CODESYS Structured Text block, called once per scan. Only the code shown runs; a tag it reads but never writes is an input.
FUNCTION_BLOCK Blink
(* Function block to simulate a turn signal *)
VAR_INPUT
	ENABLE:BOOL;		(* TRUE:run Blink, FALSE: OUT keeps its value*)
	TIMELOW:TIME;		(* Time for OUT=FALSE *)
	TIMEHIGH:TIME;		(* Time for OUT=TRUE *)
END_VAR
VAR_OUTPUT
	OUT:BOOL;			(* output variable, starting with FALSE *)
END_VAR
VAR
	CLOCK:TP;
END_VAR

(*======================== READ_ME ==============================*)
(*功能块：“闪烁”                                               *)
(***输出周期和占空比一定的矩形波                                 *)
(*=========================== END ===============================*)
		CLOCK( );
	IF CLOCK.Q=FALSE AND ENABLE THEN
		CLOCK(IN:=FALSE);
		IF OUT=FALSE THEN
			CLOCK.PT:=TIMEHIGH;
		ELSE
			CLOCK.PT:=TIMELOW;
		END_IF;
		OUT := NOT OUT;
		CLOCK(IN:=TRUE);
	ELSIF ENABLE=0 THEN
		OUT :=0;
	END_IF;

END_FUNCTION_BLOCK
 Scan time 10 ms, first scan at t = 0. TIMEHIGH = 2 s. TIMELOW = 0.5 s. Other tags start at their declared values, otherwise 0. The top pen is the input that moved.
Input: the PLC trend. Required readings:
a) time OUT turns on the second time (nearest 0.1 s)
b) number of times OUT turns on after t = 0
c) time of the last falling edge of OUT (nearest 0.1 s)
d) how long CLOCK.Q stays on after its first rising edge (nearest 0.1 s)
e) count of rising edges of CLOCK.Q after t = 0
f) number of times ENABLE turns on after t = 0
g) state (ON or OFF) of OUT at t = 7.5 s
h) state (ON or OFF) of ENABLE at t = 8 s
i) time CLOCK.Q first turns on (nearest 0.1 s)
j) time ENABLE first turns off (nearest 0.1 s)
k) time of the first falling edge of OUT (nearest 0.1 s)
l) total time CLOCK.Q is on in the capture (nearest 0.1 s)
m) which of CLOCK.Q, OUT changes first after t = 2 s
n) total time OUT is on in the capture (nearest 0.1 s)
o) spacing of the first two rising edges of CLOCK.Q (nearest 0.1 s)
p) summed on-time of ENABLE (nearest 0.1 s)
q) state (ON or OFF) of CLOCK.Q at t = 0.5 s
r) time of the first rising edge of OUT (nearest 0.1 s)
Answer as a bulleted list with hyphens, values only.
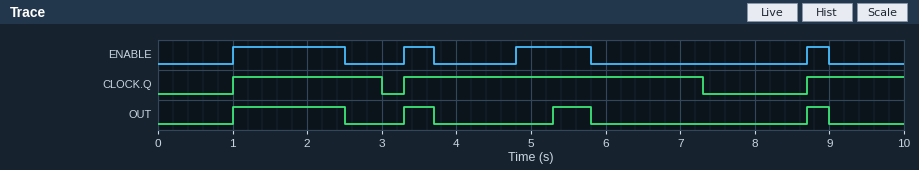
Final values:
- 3.3 s
- 4
- 9.0 s
- 2.0 s
- 3
- 4
- OFF
- OFF
- 1.0 s
- 2.5 s
- 2.5 s
- 7.3 s
- OUT
- 2.7 s
- 2.3 s
- 3.2 s
- OFF
- 1.0 s
